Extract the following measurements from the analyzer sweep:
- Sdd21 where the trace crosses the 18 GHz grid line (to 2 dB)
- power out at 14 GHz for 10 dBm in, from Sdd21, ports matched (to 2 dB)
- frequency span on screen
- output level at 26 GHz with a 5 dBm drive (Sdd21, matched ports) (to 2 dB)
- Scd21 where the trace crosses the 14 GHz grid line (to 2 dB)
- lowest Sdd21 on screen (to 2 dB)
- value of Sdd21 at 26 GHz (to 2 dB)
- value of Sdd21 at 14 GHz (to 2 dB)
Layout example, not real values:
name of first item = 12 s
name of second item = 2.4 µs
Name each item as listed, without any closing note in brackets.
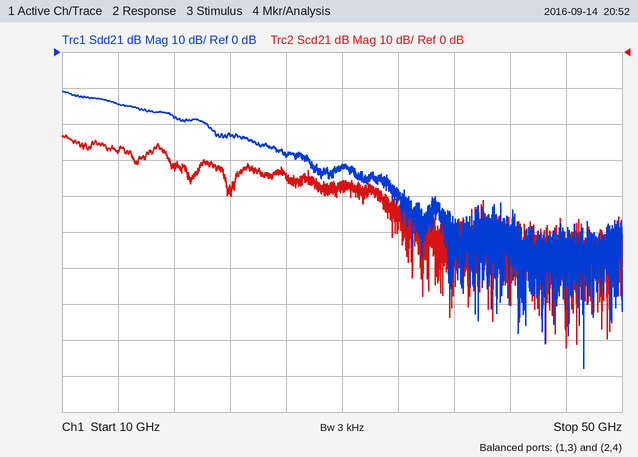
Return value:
Sdd21 where the trace crosses the 18 GHz grid line = -18 dB
power out at 14 GHz for 10 dBm in, from Sdd21, ports matched = -4 dBm
frequency span on screen = 40 GHz
output level at 26 GHz with a 5 dBm drive (Sdd21, matched ports) = -24 dBm
Scd21 where the trace crosses the 14 GHz grid line = -28 dB
lowest Sdd21 on screen = -88 dB
value of Sdd21 at 26 GHz = -28 dB
value of Sdd21 at 14 GHz = -14 dB
